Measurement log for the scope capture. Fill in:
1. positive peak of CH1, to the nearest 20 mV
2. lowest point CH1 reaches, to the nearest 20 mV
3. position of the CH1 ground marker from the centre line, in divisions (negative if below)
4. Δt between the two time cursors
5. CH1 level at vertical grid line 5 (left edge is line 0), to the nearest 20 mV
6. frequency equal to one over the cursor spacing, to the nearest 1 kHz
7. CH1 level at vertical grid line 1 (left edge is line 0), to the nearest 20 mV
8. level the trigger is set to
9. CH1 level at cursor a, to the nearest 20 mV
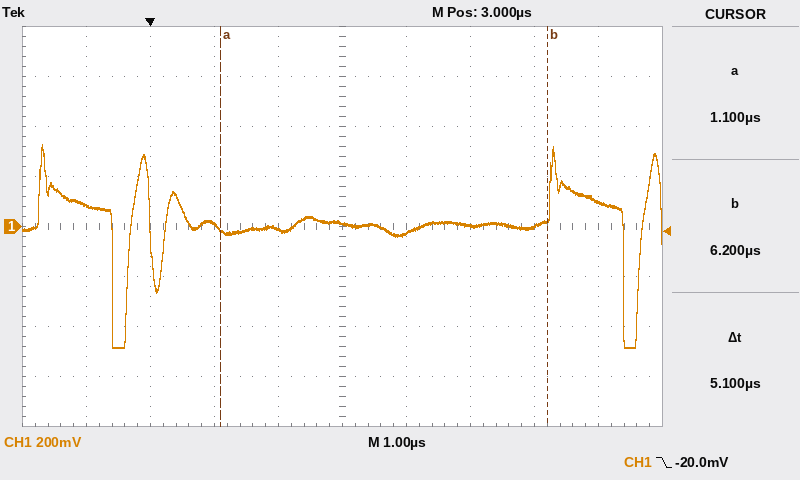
320 mV
-480 mV
0.0 div
5.1 µs
20 mV
196 kHz
80 mV
-20.0 mV
-20 mV
